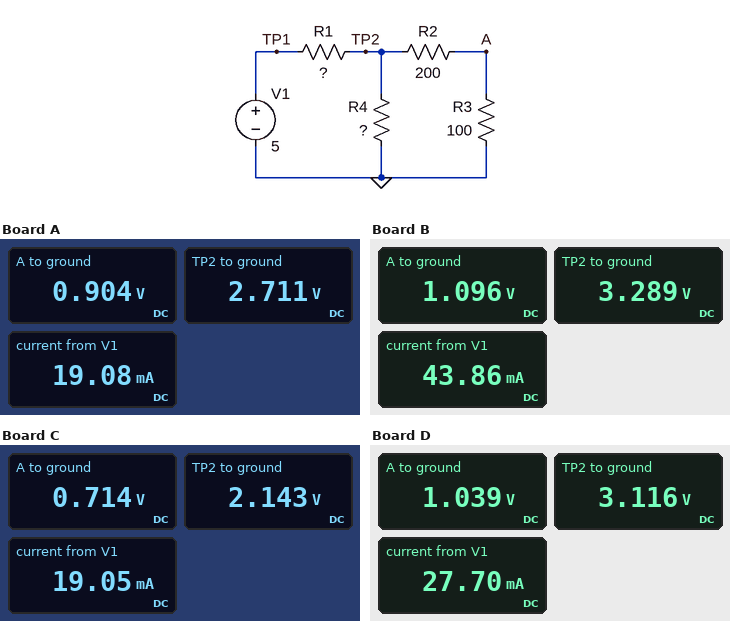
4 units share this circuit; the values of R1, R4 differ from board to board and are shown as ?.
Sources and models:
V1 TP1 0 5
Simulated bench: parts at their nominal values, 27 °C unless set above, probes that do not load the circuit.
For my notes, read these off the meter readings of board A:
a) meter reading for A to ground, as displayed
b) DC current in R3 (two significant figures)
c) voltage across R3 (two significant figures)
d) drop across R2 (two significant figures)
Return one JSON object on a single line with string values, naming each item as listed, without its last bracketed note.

{"meter reading for A to ground, as displayed": "0.904 V", "DC current in R3": "9.0 mA", "voltage across R3": "900 mV", "drop across R2": "1.8 V"}
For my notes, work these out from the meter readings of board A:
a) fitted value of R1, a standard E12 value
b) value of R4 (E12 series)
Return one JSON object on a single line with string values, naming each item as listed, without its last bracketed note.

{"fitted value of R1, a standard E12 value": "120 Ω", "value of R4": "270 Ω"}
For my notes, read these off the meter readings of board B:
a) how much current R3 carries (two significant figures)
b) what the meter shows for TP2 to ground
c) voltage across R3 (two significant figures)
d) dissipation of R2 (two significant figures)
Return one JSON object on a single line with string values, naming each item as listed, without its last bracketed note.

{"how much current R3 carries": "11 mA", "what the meter shows for TP2 to ground": "3.289 V", "voltage across R3": "1.1 V", "dissipation of R2": "24 mW"}
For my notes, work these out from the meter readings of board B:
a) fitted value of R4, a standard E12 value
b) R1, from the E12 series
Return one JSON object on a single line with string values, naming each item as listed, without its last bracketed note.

{"fitted value of R4, a standard E12 value": "100 Ω", "R1, from the E12 series": "39 Ω"}
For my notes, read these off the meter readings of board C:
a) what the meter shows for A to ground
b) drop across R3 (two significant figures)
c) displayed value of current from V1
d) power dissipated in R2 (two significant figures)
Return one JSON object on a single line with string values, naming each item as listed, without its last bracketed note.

{"what the meter shows for A to ground": "0.714 V", "drop across R3": "710 mV", "displayed value of current from V1": "19.05 mA", "power dissipated in R2": "10 mW"}
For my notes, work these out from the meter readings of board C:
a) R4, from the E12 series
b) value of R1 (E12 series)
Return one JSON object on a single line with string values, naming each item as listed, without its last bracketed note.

{"R4, from the E12 series": "180 Ω", "value of R1": "150 Ω"}
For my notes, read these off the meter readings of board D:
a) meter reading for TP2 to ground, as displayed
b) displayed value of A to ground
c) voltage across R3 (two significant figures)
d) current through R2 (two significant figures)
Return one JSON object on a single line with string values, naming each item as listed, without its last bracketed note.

{"meter reading for TP2 to ground, as displayed": "3.116 V", "displayed value of A to ground": "1.039 V", "voltage across R3": "1.0 V", "current through R2": "10 mA"}
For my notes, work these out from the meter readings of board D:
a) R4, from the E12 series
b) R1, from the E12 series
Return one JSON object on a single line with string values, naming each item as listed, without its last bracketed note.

{"R4, from the E12 series": "180 Ω", "R1, from the E12 series": "68 Ω"}
